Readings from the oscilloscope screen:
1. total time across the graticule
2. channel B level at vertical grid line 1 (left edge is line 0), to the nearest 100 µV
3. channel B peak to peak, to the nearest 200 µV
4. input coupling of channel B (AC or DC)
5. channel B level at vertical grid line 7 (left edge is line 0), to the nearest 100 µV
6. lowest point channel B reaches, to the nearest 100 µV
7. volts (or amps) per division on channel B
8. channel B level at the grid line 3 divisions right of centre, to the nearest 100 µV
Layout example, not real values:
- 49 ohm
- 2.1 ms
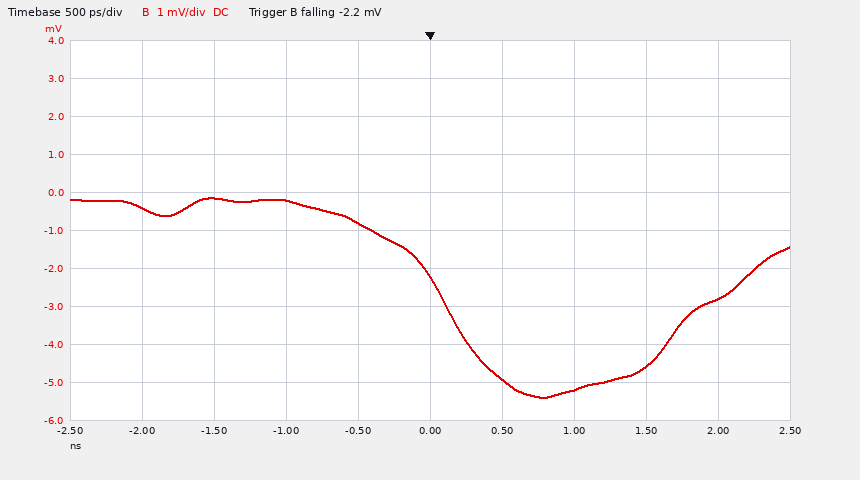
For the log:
- 5 ns
- -400 µV
- 5.2 mV
- DC
- -5.2 mV
- -5.4 mV
- 1 mV
- -4.6 mV
